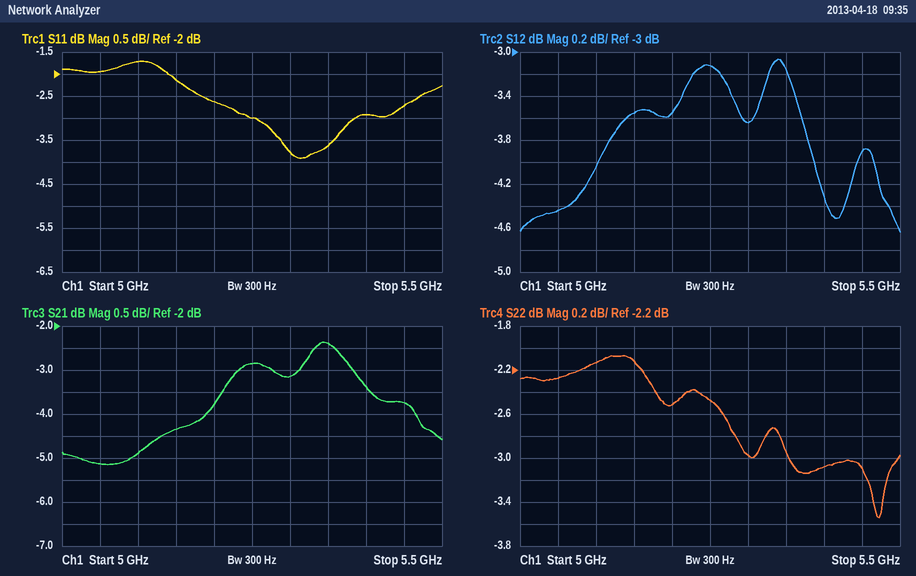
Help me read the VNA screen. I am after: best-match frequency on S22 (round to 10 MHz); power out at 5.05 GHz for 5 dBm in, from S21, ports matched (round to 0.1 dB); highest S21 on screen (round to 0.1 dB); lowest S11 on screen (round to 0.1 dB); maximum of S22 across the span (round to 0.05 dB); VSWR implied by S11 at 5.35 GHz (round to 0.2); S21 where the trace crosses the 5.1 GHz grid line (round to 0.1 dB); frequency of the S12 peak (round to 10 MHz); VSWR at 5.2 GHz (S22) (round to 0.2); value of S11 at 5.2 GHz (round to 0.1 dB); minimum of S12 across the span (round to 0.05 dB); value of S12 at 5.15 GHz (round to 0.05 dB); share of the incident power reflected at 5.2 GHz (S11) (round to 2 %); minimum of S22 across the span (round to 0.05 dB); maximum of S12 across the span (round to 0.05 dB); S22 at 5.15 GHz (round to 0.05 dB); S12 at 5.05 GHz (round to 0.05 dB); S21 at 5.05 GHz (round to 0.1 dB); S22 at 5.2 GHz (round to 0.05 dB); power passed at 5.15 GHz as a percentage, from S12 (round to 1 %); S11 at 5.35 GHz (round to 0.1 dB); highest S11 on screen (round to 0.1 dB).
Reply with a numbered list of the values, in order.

1. 5.47 GHz
2. -0.1 dBm
3. -2.4 dB
4. -3.9 dB
5. -2.05 dB
6. 4.8
7. -4.9 dB
8. 5.34 GHz
9. 7.0
10. -2.6 dB
11. -4.65 dB
12. -3.55 dB
13. 54 %
14. -3.55 dB
15. -3.05 dB
16. -2.10 dB
17. -4.45 dB
18. -5.1 dB
19. -2.50 dB
20. 44 %
21. -3.6 dB
22. -1.7 dB
